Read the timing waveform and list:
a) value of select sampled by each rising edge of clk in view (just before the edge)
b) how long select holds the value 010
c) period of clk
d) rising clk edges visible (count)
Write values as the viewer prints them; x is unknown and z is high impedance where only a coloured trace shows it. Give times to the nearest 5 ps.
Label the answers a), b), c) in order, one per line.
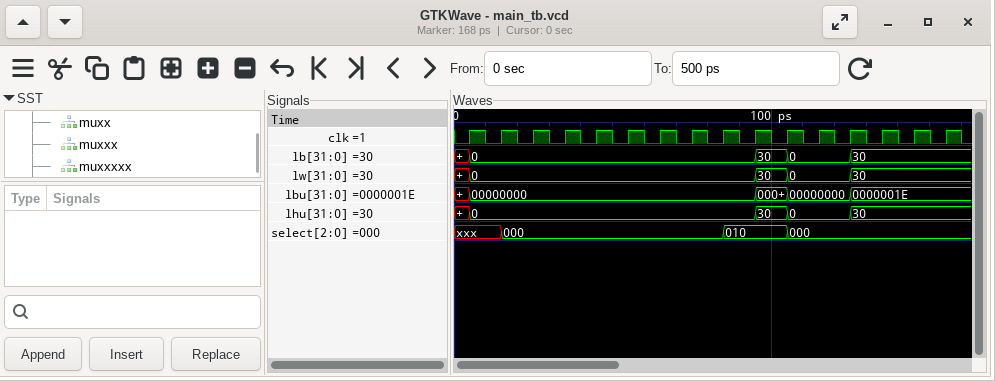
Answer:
a) xxx, xxx, 000, 000, 000, 000, 000, 000, 000, 010, 010, 000, 000, 000, 000, 000
b) 20 ps
c) 10 ps
d) 16
